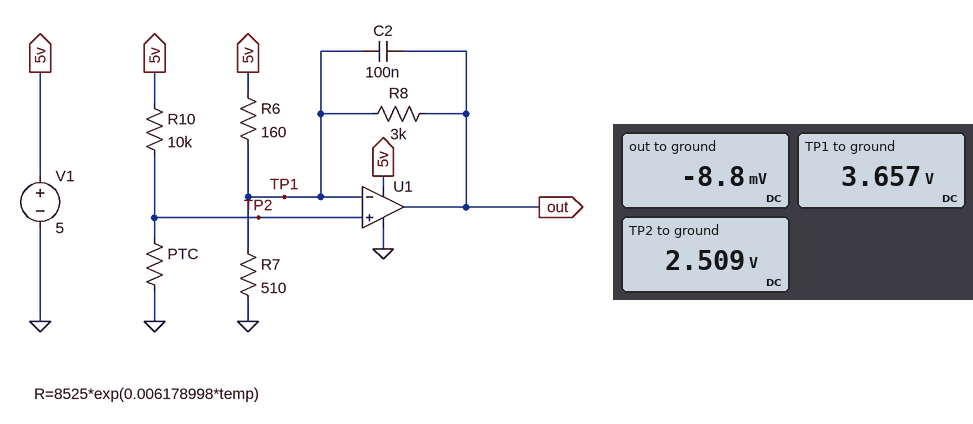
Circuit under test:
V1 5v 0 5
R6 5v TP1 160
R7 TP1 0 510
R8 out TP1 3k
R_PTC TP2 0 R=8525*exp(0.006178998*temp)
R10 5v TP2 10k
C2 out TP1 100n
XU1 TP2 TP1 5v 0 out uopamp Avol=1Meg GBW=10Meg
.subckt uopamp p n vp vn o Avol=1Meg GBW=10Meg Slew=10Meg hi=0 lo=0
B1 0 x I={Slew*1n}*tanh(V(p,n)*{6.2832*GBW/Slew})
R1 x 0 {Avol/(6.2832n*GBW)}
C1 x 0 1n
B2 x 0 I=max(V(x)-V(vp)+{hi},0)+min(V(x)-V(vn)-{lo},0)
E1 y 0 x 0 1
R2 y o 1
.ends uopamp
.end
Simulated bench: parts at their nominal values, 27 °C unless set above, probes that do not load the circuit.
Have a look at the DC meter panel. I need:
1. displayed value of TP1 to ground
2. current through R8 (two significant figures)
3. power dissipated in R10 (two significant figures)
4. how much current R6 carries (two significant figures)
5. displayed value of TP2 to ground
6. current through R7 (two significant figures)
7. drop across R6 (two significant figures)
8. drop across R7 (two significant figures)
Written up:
3.657 V
1.2 mA
620 µW
8.4 mA
2.509 V
7.2 mA
1.3 V
3.7 V
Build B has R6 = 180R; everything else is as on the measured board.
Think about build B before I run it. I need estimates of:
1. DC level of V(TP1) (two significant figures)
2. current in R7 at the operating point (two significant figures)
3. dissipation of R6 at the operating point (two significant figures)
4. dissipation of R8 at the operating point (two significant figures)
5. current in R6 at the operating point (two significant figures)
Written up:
3.5 V
6.9 mA
12 mW
4.2 mW
8.1 mA
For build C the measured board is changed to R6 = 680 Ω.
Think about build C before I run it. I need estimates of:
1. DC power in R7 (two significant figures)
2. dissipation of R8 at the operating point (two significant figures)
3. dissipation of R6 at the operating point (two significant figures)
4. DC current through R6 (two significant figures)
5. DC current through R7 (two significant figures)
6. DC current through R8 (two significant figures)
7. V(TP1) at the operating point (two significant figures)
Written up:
11 mW
2.3 mW
10 mW
3.8 mA
4.7 mA
870 µA
2.4 V
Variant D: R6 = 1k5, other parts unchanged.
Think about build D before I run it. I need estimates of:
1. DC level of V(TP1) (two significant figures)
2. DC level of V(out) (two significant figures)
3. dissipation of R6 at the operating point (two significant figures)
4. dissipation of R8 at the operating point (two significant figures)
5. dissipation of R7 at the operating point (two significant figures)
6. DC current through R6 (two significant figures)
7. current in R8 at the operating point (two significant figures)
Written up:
1.7 V
5.0 V
7.3 mW
3.7 mW
5.6 mW
2.2 mA
1.1 mA
